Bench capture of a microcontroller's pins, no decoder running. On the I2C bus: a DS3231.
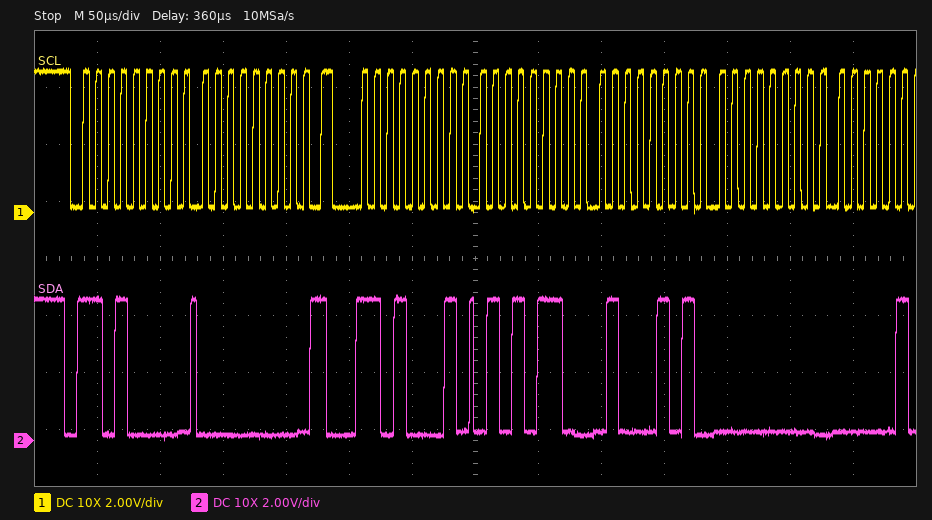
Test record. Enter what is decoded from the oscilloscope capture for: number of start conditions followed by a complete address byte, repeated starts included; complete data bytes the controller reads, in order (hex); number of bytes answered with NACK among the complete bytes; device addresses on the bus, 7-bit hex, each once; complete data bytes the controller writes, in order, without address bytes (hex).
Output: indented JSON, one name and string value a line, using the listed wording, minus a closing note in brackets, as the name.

{
  "number of start conditions followed by a complete address byte, repeated starts included": "2",
  "complete data bytes the controller reads, in order": "56 45 00",
  "number of bytes answered with NACK among the complete bytes": "0",
  "device addresses on the bus, 7-bit hex, each once": "0x68",
  "complete data bytes the controller writes, in order, without address bytes": "00"
}
